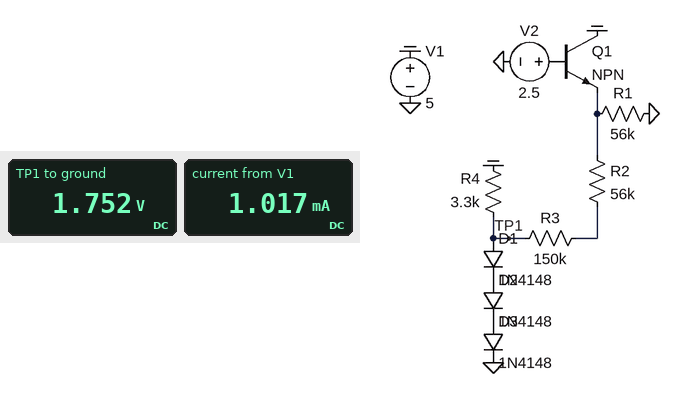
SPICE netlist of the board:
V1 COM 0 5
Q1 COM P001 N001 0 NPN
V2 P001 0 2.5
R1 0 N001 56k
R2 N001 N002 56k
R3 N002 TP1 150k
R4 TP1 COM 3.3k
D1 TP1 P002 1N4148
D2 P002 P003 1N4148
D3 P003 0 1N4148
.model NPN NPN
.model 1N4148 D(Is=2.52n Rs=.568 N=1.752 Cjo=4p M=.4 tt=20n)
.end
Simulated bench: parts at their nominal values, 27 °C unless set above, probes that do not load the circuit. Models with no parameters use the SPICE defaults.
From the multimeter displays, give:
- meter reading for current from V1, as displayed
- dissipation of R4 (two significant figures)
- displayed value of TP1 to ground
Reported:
1.017 mA
3.2 mW
1.752 V
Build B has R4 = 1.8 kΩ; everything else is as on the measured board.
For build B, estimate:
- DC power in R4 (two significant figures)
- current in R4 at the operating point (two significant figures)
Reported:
5.6 mW
1.8 mA
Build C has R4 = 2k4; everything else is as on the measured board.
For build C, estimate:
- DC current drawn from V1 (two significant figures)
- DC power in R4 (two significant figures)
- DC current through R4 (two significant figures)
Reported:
1.4 mA
4.3 mW
1.3 mA
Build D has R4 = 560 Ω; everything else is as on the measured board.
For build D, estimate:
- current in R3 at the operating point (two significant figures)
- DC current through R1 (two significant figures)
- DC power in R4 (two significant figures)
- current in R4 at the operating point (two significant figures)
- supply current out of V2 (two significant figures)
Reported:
850 nA
32 µA
16 mW
5.4 mA
310 nA
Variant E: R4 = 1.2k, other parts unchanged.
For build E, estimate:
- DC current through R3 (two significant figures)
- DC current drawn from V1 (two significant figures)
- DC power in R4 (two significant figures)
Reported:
350 nA
2.6 mA
8.1 mW
